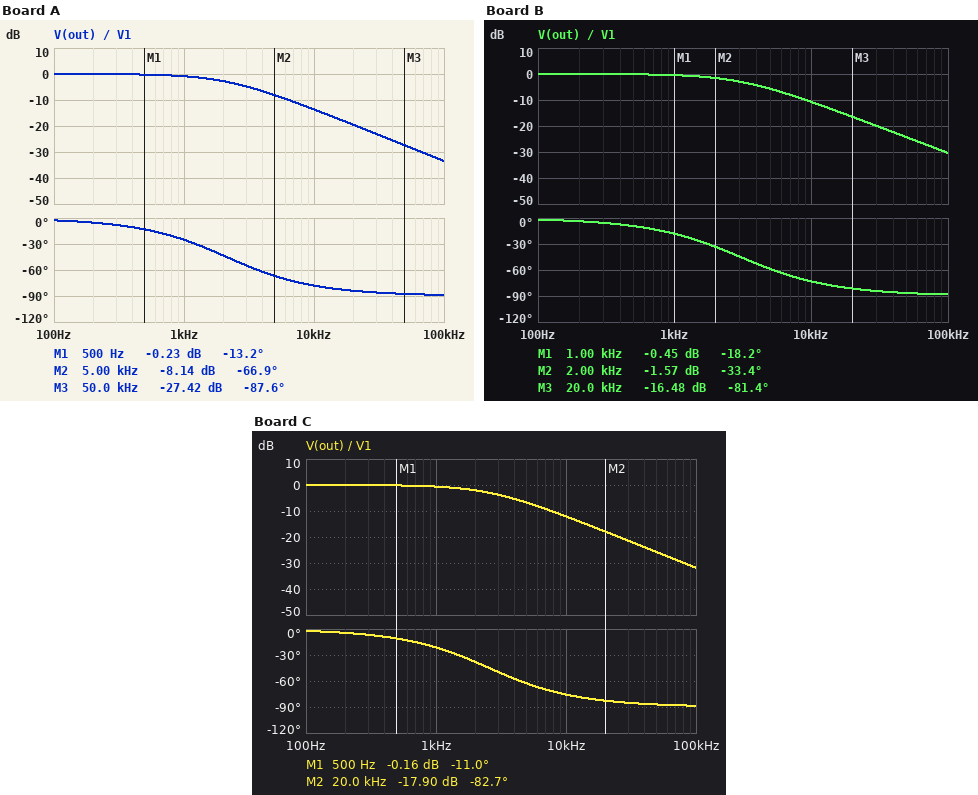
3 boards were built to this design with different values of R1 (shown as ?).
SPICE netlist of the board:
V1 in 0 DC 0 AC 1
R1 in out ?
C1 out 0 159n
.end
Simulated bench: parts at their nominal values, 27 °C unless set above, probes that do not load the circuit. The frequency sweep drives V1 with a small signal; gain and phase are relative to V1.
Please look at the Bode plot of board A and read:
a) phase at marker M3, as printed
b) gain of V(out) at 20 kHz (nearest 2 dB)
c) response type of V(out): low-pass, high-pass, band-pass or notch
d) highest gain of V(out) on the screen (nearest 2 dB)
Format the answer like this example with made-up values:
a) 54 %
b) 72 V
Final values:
a) -87.6 deg
b) -20 dB
c) low-pass
d) 0 dB
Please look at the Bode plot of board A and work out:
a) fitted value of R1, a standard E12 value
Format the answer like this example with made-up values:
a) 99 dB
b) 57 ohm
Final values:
a) 470 Ω
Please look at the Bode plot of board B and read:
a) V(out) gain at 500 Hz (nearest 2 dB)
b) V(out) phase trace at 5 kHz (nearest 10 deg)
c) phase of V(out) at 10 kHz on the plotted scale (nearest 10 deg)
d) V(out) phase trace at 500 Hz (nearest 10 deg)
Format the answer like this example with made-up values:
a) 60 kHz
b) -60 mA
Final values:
a) 0 dB
b) -60 deg
c) -70 deg
d) -10 deg
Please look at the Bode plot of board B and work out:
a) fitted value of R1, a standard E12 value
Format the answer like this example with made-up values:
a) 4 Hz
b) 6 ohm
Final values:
a) 330 Ω
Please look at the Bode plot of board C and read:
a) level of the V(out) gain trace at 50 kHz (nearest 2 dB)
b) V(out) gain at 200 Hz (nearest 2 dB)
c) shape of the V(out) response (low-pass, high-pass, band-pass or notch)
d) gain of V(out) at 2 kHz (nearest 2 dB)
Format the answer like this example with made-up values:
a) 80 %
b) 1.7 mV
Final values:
a) -26 dB
b) 0 dB
c) low-pass
d) -2 dB
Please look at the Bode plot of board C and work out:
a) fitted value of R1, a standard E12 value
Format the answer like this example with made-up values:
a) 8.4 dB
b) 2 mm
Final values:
a) 390 Ω
